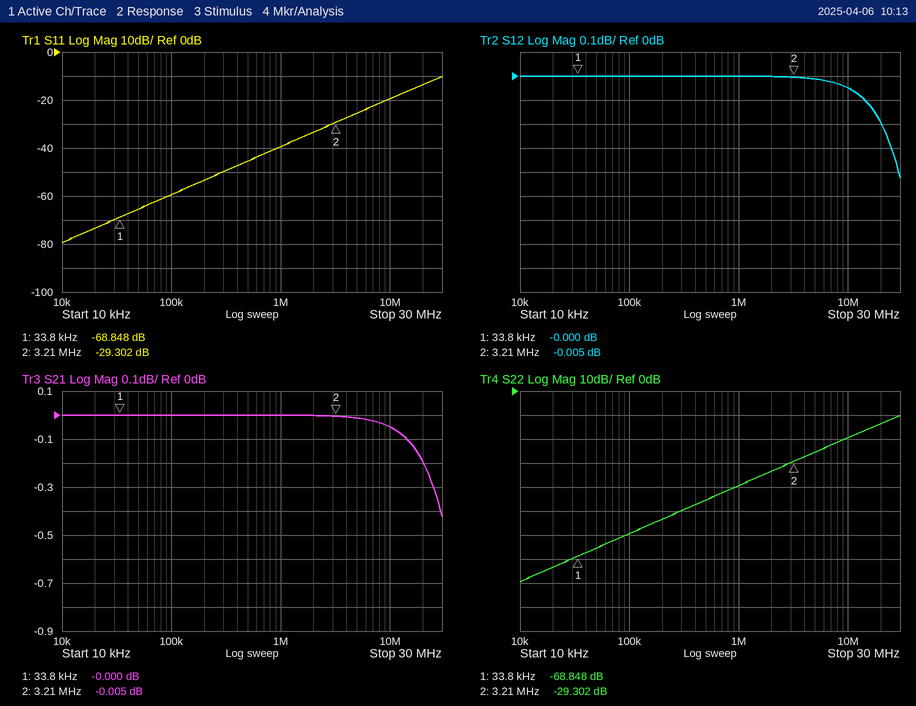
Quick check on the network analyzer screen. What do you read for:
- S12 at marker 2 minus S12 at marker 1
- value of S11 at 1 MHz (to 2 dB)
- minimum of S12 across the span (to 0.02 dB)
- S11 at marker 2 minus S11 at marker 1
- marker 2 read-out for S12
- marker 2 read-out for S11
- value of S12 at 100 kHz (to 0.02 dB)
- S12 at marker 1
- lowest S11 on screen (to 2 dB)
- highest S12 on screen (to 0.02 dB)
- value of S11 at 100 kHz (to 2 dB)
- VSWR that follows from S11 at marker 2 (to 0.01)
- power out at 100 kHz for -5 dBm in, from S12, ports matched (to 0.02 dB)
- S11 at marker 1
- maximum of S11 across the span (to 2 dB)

-0.005 dB
-40 dB
-0.42 dB
39.546 dB
-0.005 dB
-29.302 dB
0.00 dB
-0.000 dB
-80 dB
0.00 dB
-60 dB
1.07
-5.00 dBm
-68.848 dB
-10 dB
